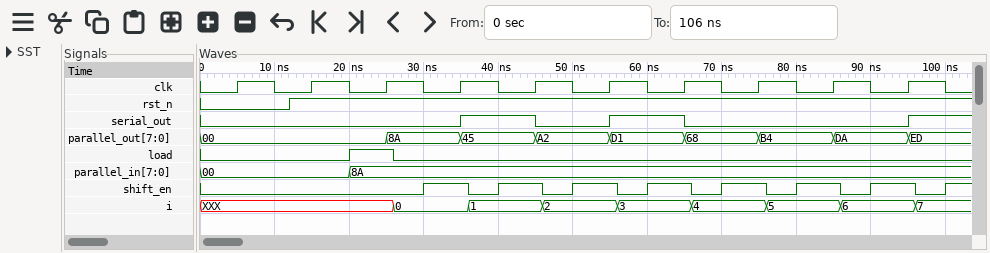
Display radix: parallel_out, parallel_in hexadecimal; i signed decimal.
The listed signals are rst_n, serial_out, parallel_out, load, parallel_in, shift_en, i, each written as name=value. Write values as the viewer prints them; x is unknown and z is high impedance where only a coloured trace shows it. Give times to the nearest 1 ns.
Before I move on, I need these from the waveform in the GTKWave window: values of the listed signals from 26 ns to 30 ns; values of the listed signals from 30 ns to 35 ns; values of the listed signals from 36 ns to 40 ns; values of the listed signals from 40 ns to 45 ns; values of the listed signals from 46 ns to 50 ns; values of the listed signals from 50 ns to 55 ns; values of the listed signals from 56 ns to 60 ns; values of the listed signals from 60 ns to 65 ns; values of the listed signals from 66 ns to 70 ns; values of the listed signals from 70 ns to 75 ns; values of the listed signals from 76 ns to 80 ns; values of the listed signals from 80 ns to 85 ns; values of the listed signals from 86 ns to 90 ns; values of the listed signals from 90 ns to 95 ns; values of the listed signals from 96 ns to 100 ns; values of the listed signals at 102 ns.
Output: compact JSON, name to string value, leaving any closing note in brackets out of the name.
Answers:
{"values of the listed signals from 26 ns to 30 ns": "rst_n=1, serial_out=0, parallel_out=8A, load=0, parallel_in=8A, shift_en=0, i=0", "values of the listed signals from 30 ns to 35 ns": "rst_n=1, serial_out=0, parallel_out=8A, load=0, parallel_in=8A, shift_en=1, i=0", "values of the listed signals from 36 ns to 40 ns": "rst_n=1, serial_out=1, parallel_out=45, load=0, parallel_in=8A, shift_en=0, i=1", "values of the listed signals from 40 ns to 45 ns": "rst_n=1, serial_out=1, parallel_out=45, load=0, parallel_in=8A, shift_en=1, i=1", "values of the listed signals from 46 ns to 50 ns": "rst_n=1, serial_out=0, parallel_out=A2, load=0, parallel_in=8A, shift_en=0, i=2", "values of the listed signals from 50 ns to 55 ns": "rst_n=1, serial_out=0, parallel_out=A2, load=0, parallel_in=8A, shift_en=1, i=2", "values of the listed signals from 56 ns to 60 ns": "rst_n=1, serial_out=1, parallel_out=D1, load=0, parallel_in=8A, shift_en=0, i=3", "values of the listed signals from 60 ns to 65 ns": "rst_n=1, serial_out=1, parallel_out=D1, load=0, parallel_in=8A, shift_en=1, i=3", "values of the listed signals from 66 ns to 70 ns": "rst_n=1, serial_out=0, parallel_out=68, load=0, parallel_in=8A, shift_en=0, i=4", "values of the listed signals from 70 ns to 75 ns": "rst_n=1, serial_out=0, parallel_out=68, load=0, parallel_in=8A, shift_en=1, i=4", "values of the listed signals from 76 ns to 80 ns": "rst_n=1, serial_out=0, parallel_out=B4, load=0, parallel_in=8A, shift_en=0, i=5", "values of the listed signals from 80 ns to 85 ns": "rst_n=1, serial_out=0, parallel_out=B4, load=0, parallel_in=8A, shift_en=1, i=5", "values of the listed signals from 86 ns to 90 ns": "rst_n=1, serial_out=0, parallel_out=DA, load=0, parallel_in=8A, shift_en=0, i=6", "values of the listed signals from 90 ns to 95 ns": "rst_n=1, serial_out=0, parallel_out=DA, load=0, parallel_in=8A, shift_en=1, i=6", "values of the listed signals from 96 ns to 100 ns": "rst_n=1, serial_out=1, parallel_out=ED, load=0, parallel_in=8A, shift_en=0, i=7", "values of the listed signals at 102 ns": "rst_n=1, serial_out=1, parallel_out=ED, load=0, parallel_in=8A, shift_en=1, i=7"}
